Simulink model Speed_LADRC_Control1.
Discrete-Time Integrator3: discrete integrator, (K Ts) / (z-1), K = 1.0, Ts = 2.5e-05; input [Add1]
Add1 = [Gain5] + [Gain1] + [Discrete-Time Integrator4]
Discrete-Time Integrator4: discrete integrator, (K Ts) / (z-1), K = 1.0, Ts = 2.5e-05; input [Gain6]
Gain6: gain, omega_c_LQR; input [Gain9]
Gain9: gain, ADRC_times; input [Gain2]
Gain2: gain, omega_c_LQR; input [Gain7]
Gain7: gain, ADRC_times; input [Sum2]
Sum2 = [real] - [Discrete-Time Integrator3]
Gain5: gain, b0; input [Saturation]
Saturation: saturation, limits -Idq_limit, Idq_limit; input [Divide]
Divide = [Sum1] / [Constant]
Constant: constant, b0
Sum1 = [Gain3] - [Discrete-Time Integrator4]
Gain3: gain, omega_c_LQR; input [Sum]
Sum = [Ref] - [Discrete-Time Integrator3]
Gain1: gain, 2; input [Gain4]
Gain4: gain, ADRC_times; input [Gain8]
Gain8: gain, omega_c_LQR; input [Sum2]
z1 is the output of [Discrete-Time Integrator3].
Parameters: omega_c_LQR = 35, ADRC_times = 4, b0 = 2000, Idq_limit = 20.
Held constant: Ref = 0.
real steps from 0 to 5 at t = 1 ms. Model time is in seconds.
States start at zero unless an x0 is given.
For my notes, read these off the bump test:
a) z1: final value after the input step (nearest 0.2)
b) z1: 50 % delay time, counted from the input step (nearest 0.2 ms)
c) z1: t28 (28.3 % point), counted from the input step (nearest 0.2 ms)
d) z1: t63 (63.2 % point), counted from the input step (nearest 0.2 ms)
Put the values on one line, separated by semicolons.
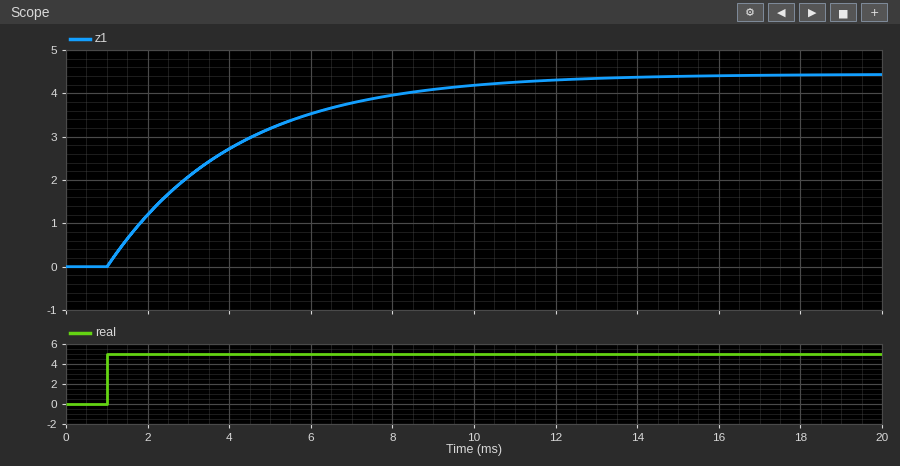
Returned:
4.4; 2.2 ms; 1.0 ms; 3.2 ms
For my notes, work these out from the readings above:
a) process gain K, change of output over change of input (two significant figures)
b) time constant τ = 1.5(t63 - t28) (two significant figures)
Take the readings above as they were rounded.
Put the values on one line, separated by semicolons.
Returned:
0.88; 3.3 ms
